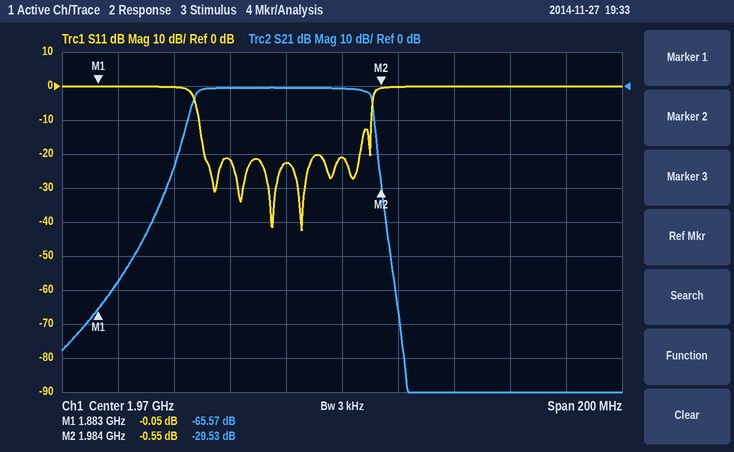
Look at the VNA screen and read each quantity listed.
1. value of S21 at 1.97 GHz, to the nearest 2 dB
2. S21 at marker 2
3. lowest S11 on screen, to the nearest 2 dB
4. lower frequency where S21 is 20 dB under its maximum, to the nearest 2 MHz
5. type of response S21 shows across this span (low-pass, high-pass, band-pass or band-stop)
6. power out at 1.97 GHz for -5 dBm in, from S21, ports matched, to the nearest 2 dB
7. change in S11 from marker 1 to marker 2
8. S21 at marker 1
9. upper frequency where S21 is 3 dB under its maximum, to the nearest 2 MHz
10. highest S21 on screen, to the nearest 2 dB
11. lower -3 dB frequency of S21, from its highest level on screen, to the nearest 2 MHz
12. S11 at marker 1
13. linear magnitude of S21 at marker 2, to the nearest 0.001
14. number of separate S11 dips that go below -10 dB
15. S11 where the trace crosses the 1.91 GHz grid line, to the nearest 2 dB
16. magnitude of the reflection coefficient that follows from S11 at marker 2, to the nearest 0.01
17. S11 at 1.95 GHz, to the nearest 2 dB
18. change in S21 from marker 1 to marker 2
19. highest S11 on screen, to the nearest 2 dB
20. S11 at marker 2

0 dB
-29.53 dB
-42 dB
1.912 GHz
band-pass
-6 dBm
-0.50 dB
-65.57 dB
1.980 GHz
0 dB
1.918 GHz
-0.05 dB
0.033
7
0 dB
0.94
-22 dB
36.04 dB
0 dB
-0.55 dB
